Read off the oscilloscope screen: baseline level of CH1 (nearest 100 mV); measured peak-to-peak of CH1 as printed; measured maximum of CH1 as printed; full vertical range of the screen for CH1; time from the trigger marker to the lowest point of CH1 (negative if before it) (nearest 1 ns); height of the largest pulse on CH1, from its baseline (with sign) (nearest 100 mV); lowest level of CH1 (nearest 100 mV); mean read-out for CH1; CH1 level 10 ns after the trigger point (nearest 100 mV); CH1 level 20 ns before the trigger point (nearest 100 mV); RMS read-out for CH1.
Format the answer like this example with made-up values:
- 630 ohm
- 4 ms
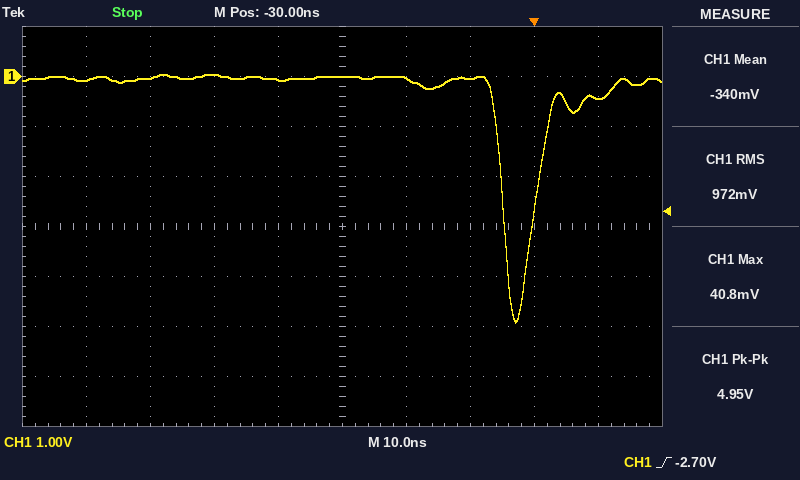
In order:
- 0.0 V
- 4.95 V
- 40.8 mV
- 8 V
- -3 ns
- -4.9 V
- -4.9 V
- -340 mV
- -400 mV
- 0.0 V
- 972 mV
